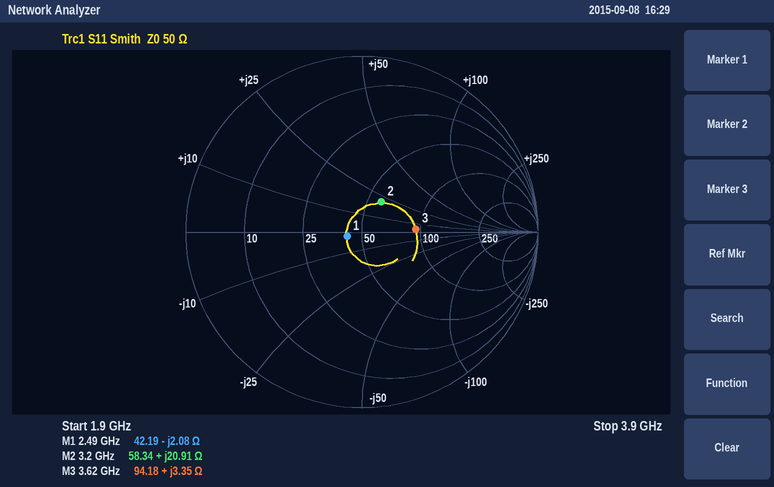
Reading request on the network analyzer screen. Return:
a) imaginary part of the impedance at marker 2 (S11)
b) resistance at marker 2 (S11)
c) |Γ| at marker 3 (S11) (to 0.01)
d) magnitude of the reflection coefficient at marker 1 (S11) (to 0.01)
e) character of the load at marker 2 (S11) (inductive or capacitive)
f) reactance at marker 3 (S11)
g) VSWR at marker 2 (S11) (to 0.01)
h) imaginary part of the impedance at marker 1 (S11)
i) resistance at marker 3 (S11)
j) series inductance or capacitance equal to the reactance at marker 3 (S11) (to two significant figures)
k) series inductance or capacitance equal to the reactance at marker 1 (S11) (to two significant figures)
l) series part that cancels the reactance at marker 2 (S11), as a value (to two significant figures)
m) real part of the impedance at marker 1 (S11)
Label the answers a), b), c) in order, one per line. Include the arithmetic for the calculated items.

a) +20.91 Ω
b) 58.34 Ω
c) 0.31
d) 0.09
e) inductive
f) +3.35 Ω
g) 1.51
h) -2.08 Ω
i) 94.18 Ω
j) L = 3.35 Ω/(2π × 3.62 GHz) ≈ 147 pH, so 150 pH to two significant figures
k) C = 1/(2π × 2.49 GHz × 2.08 Ω) ≈ 31 pF
l) C = 1/(2π × 3.2 GHz × 20.91 Ω) ≈ 2.4 pF
m) 42.19 Ω
